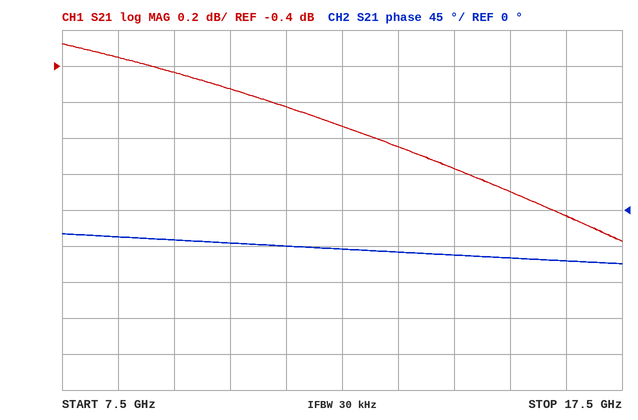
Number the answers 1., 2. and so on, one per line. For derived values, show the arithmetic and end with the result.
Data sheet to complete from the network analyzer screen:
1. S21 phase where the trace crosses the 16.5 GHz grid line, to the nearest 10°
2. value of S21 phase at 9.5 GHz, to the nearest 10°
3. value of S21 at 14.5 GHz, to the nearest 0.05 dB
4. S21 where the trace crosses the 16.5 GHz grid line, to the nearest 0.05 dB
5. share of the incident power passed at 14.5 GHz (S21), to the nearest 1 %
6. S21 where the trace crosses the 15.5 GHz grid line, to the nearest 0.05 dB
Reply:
1. -60°
2. -40°
3. -0.95 dB
4. -1.25 dB
5. 10^(-0.95/10) ≈ 80 %
6. -1.10 dB
